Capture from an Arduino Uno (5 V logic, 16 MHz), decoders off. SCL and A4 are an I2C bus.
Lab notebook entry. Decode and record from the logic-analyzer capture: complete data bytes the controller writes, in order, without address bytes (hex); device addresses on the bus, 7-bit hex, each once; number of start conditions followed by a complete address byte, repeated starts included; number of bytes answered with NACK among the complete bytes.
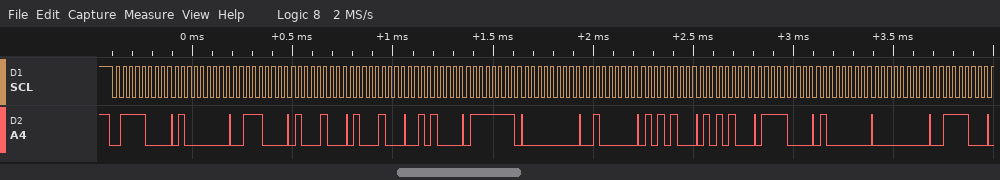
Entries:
40 38 44 44 28 7F 00 20 54 54 78 40 00 3C
0x3C
1
0
